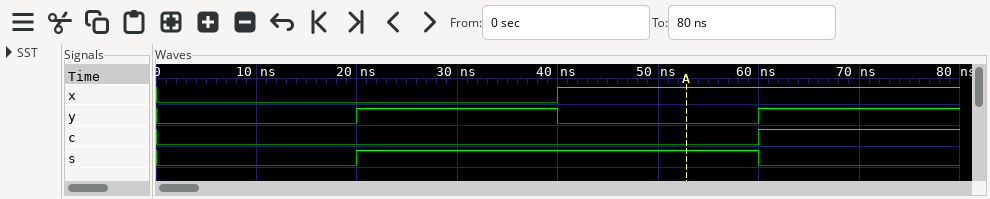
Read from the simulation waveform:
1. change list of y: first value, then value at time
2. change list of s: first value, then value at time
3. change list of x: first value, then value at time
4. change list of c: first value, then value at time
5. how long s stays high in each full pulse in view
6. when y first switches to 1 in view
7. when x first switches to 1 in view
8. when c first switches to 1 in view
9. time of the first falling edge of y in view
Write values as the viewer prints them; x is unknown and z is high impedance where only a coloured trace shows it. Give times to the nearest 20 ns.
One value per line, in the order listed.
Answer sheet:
0, 1 at 20 ns, 0 at 40 ns, 1 at 60 ns
0, 1 at 20 ns, 0 at 60 ns
0, 1 at 40 ns
0, 1 at 60 ns
40 ns
20 ns
40 ns
60 ns
40 ns
